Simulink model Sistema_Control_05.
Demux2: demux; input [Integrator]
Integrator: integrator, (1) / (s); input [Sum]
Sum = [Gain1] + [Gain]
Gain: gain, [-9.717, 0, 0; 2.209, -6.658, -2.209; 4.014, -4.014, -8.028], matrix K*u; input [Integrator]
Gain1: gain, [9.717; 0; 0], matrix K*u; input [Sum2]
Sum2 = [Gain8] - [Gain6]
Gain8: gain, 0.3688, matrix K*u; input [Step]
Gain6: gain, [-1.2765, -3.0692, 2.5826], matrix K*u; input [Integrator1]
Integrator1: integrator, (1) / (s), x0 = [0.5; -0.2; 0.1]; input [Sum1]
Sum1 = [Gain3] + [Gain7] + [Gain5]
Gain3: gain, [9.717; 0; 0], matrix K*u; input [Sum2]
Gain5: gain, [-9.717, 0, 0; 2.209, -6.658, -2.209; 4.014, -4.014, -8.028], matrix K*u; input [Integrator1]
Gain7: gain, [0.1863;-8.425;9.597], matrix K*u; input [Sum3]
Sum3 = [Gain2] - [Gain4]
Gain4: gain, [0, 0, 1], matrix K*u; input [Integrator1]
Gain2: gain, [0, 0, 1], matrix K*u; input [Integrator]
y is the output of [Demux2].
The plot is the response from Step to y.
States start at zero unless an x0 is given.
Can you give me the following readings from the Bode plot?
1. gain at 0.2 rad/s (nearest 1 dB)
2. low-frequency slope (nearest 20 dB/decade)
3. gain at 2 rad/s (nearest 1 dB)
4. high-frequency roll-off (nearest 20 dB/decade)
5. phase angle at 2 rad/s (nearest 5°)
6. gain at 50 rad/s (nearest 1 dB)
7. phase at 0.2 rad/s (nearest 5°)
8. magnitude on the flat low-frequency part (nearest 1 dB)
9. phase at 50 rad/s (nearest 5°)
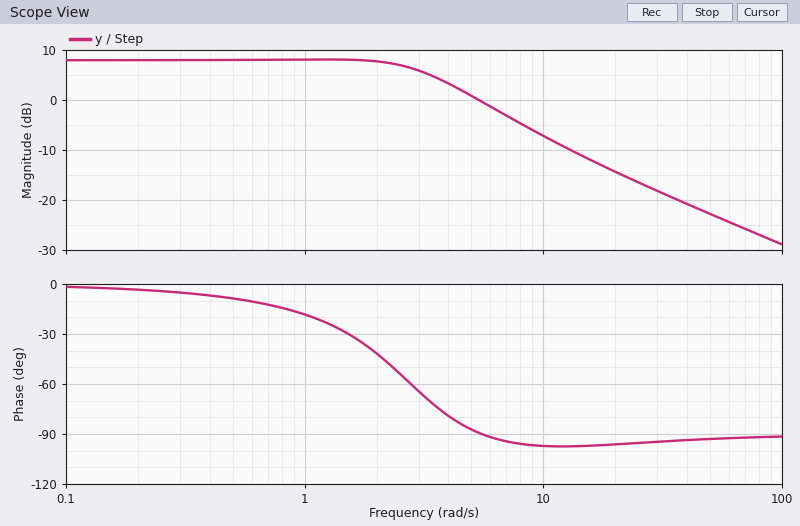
8 dB
0 dB/decade
8 dB
-20 dB/decade
-40°
-23 dB
-5°
8 dB
-95°
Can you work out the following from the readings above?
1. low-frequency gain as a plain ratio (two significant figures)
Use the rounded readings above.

2.5
